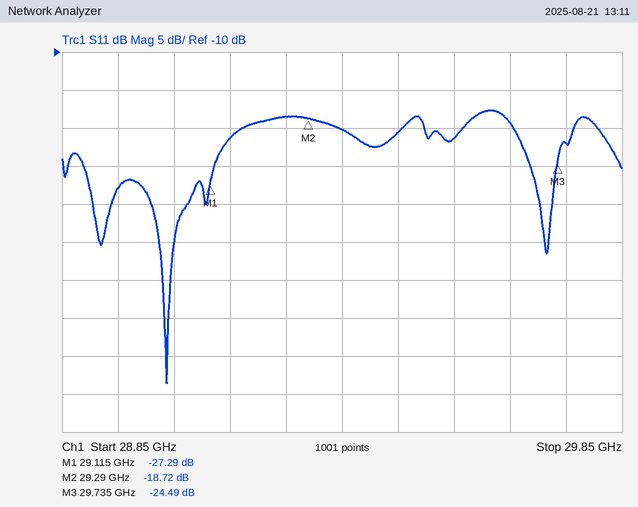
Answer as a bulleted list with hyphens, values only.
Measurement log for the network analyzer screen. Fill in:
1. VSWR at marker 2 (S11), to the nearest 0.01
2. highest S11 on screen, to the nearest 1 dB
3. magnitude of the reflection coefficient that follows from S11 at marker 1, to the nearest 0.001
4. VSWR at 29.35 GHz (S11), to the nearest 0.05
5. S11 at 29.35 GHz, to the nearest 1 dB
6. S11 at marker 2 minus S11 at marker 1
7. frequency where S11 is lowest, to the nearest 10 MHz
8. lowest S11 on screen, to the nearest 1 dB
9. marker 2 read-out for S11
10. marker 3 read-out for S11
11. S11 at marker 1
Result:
- 1.26
- -18 dB
- 0.043
- 1.20
- -20 dB
- 8.57 dB
- 29.04 GHz
- -54 dB
- -18.72 dB
- -24.49 dB
- -27.29 dB
